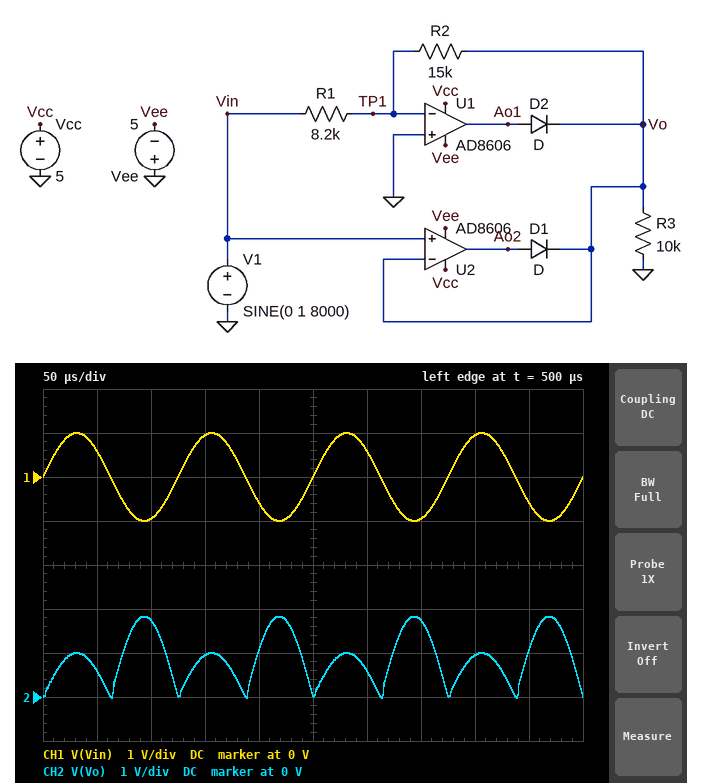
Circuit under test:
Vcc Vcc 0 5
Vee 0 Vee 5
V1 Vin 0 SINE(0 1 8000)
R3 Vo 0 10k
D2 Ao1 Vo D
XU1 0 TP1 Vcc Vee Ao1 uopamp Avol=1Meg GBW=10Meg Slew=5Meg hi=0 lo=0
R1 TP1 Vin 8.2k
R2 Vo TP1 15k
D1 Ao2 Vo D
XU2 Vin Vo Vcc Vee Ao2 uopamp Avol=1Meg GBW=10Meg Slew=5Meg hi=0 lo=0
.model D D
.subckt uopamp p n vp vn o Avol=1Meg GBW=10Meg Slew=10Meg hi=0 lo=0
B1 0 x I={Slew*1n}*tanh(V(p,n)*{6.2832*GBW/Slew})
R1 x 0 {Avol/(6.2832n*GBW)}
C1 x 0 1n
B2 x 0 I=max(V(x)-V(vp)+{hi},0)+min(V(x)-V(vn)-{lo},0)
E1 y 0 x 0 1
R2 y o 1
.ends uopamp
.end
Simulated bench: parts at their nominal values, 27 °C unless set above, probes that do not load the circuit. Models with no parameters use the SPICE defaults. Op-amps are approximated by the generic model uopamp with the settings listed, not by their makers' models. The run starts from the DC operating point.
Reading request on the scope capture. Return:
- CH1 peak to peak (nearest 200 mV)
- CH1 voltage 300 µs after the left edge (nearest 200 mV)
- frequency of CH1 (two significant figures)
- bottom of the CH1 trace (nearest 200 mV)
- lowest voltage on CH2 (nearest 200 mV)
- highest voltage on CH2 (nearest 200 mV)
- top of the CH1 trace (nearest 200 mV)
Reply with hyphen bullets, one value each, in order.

- 2.0 V
- 600 mV
- 8.0 kHz
- -1.0 V
- 0 V
- 1.8 V
- 1.0 V
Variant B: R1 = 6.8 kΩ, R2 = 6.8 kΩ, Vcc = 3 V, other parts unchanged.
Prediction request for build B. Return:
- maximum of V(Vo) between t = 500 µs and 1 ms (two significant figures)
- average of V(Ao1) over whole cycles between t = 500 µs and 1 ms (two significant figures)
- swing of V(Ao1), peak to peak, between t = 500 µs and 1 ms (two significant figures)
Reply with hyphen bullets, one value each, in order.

- 1.0 V
- -1.9 V
- 6.6 V
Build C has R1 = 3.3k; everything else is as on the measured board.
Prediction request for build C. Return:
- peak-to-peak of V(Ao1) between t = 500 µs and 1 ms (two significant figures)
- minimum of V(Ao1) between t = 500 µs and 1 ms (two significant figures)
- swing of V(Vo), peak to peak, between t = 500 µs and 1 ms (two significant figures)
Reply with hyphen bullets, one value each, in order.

- 10 V
- -5.0 V
- 4.4 V
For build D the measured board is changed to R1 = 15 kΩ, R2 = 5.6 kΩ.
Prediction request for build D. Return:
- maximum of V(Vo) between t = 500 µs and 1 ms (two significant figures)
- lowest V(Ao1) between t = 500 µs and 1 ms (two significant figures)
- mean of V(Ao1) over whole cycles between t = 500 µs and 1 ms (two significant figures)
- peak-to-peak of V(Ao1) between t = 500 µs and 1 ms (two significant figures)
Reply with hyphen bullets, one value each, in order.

- 1.0 V
- -5.0 V
- -2.1 V
- 6.0 V
